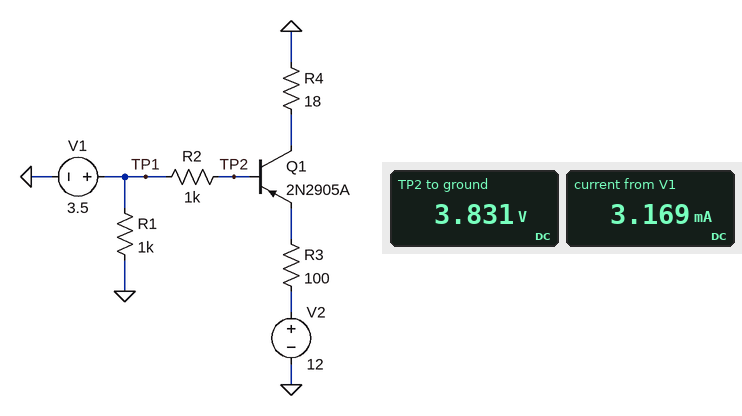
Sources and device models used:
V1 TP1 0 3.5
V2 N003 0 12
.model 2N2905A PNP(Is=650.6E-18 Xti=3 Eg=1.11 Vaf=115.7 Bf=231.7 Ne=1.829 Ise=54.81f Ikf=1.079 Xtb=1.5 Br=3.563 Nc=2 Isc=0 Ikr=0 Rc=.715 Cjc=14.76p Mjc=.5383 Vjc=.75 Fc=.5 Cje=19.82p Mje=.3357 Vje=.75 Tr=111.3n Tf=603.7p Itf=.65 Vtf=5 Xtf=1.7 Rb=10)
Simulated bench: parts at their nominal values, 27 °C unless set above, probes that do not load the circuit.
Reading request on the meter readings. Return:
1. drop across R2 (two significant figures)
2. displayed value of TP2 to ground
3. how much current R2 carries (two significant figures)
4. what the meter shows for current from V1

330 mV
3.831 V
330 µA
3.169 mA
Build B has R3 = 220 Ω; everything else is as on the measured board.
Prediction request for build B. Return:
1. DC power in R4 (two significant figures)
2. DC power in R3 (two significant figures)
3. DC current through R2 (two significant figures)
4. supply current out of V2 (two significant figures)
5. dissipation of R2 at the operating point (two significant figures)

21 mW
260 mW
150 µA
34 mA
22 µW
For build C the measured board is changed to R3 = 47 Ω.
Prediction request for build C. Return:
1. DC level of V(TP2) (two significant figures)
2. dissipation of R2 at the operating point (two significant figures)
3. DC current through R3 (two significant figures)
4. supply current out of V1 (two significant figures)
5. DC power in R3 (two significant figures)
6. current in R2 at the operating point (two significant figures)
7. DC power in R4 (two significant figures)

4.2 V
510 µW
150 mA
2.8 mA
1.0 W
710 µA
390 mW
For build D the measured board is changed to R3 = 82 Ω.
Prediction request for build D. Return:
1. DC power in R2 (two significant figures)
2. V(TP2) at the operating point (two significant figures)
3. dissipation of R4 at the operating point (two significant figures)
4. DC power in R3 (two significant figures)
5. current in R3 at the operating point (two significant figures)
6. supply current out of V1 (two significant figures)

160 µW
3.9 V
140 mW
640 mW
88 mA
3.1 mA
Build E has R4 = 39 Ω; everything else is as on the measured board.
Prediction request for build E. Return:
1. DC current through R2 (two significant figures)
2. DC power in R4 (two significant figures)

340 µA
210 mW
